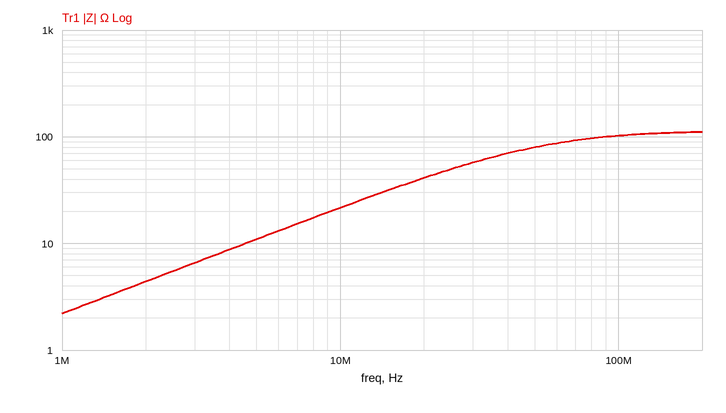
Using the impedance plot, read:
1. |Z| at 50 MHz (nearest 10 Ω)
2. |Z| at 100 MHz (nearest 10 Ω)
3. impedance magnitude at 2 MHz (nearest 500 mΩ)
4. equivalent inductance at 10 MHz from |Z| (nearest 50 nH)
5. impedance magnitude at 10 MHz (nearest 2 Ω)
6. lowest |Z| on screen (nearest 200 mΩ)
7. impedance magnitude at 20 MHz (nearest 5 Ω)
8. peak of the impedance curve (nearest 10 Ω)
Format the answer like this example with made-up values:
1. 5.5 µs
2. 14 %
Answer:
1. 80 Ω
2. 100 Ω
3. 4.5 Ω
4. 350 nH
5. 22 Ω
6. 2.2 Ω
7. 40 Ω
8. 110 Ω
